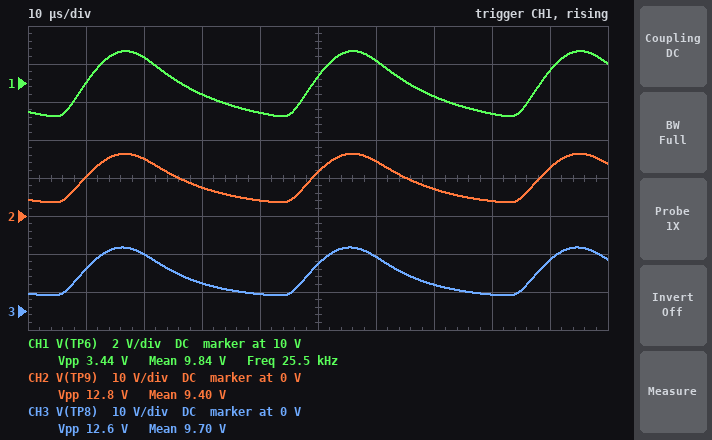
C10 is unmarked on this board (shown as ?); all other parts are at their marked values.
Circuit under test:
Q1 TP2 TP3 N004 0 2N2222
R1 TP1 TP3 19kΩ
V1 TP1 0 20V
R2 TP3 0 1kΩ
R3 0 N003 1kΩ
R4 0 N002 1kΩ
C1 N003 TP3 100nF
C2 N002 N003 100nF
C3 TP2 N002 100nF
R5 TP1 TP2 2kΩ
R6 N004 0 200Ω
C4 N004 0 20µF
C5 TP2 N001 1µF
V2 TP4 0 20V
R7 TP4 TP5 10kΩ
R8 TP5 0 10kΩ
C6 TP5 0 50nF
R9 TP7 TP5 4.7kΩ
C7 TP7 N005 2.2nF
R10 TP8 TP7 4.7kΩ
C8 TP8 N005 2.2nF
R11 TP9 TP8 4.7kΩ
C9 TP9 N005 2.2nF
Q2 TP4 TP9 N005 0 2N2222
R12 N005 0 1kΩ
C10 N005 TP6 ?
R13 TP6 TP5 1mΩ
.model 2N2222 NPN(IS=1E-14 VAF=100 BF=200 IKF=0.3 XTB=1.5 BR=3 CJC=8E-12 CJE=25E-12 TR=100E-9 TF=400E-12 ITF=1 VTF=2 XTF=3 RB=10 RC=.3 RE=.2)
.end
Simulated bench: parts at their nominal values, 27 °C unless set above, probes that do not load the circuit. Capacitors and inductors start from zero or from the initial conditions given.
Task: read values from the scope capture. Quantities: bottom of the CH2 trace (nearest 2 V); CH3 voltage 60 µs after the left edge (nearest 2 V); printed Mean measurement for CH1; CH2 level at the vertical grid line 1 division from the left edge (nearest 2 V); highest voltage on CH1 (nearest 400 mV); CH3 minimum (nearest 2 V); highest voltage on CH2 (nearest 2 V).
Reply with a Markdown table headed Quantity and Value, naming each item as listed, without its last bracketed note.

| Quantity | Value |
|---|---|
| bottom of the CH2 trace | 4 V |
| CH3 voltage 60 µs after the left edge | 14 V |
| printed Mean measurement for CH1 | 9.84 V |
| CH2 level at the vertical grid line 1 division from the left edge | 10 V |
| highest voltage on CH1 | 11.6 V |
| CH3 minimum | 4 V |
| highest voltage on CH2 | 16 V |
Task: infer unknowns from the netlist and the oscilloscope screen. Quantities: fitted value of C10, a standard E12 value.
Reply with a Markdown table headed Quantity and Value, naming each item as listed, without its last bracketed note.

| Quantity | Value |
|---|---|
| fitted value of C10, a standard E12 value | 18 nF |
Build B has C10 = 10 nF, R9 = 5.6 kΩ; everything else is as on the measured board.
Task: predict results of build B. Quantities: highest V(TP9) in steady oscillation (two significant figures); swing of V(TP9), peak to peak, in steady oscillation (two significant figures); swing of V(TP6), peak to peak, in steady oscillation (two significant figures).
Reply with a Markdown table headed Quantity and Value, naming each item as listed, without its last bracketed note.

| Quantity | Value |
|---|---|
| highest V(TP9) in steady oscillation | 20 V |
| swing of V(TP9), peak to peak, in steady oscillation | 18 V |
| swing of V(TP6), peak to peak, in steady oscillation | 3.1 V |
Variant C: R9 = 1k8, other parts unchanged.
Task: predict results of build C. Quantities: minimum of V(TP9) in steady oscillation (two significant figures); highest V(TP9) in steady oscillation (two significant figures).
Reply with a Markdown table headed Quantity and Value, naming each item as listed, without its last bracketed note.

| Quantity | Value |
|---|---|
| minimum of V(TP9) in steady oscillation | 3.9 V |
| highest V(TP9) in steady oscillation | 17 V |
